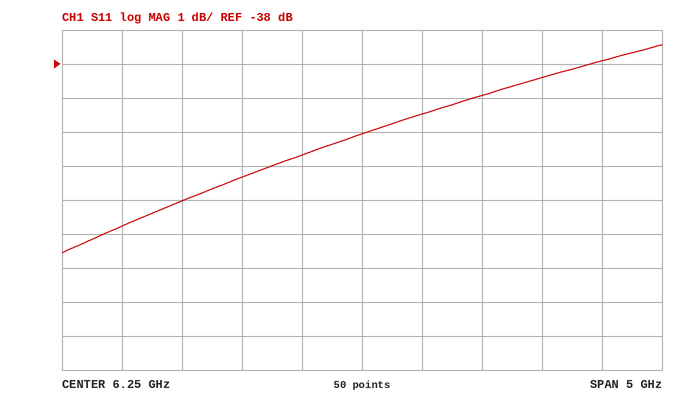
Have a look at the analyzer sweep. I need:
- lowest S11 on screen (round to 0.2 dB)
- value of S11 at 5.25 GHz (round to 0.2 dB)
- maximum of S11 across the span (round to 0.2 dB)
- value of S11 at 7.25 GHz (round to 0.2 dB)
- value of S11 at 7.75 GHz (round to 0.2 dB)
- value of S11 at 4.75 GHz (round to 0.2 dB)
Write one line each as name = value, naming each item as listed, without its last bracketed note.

lowest S11 on screen = -43.6 dB
value of S11 at 5.25 GHz = -41.4 dB
maximum of S11 across the span = -37.4 dB
value of S11 at 7.25 GHz = -39.0 dB
value of S11 at 7.75 GHz = -38.4 dB
value of S11 at 4.75 GHz = -42.0 dB
